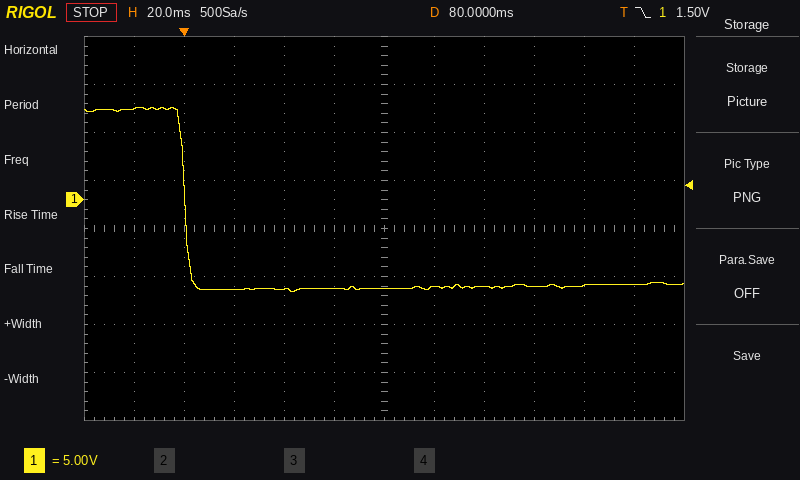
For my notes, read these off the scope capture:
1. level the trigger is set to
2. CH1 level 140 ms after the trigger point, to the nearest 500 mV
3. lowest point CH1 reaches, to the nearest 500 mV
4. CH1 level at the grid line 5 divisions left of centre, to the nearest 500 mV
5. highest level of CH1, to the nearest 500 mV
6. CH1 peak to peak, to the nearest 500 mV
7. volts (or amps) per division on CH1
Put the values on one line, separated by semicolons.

1.50 V; -9.0 V; -9.5 V; 9.5 V; 9.5 V; 19.0 V; 5 V
